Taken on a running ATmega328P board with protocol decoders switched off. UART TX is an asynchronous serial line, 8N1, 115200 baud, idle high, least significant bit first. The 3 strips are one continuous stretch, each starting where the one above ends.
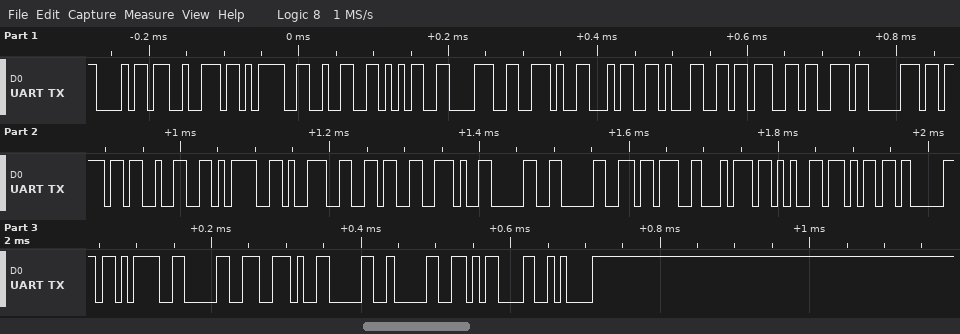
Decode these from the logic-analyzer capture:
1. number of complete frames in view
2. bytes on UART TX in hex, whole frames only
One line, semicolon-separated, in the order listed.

32; 0x68 0x72 0x3D 0x32 0x35 0x38 0x2E 0x34 0x31 0x3B 0x73 0x70 0x6F 0x32 0x3D 0x39 0x36 0x2E 0x30 0x30 0x3B 0x74 0x65 0x6D 0x70 0x3D 0x30 0x2E 0x30 0x30 0x0D 0x0A
